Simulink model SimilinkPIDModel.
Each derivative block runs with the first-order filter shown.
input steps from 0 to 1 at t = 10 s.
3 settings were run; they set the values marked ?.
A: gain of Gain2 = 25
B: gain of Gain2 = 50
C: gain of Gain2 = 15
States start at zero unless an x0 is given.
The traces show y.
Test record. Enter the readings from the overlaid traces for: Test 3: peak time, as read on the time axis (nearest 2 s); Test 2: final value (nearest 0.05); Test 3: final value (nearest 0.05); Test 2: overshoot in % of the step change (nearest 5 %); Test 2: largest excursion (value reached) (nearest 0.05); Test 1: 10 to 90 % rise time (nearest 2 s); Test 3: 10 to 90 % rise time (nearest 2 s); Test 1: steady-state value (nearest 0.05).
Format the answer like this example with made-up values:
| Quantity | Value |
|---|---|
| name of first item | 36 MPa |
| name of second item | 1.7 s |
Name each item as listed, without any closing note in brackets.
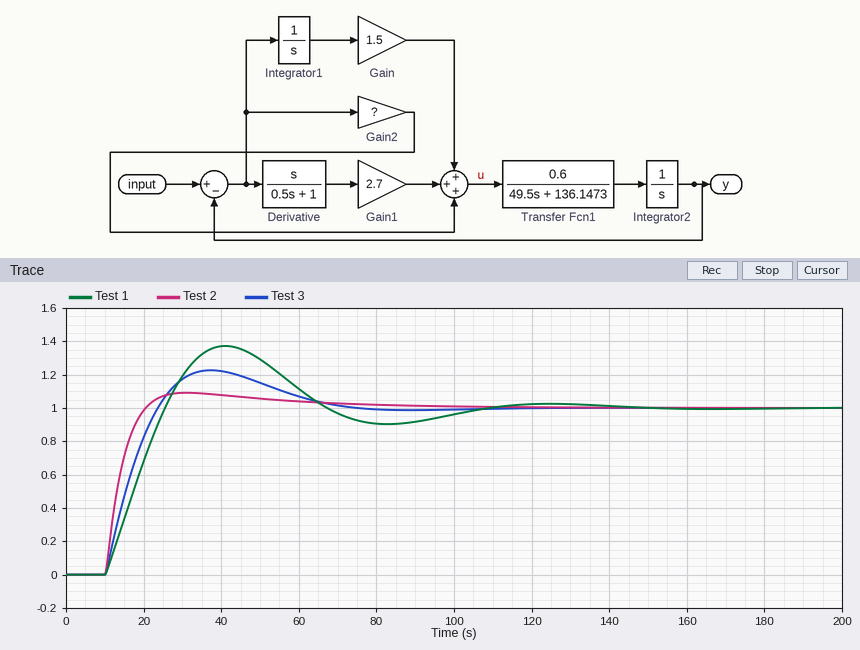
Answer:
| Quantity | Value |
|---|---|
| Test 3: peak time, as read on the time axis | 38 s |
| Test 2: final value | 1.00 |
| Test 3: final value | 1.00 |
| Test 2: overshoot in % of the step change | 10 % |
| Test 2: largest excursion (value reached) | 1.10 |
| Test 1: 10 to 90 % rise time | 12 s |
| Test 3: 10 to 90 % rise time | 10 s |
| Test 1: steady-state value | 1.00 |
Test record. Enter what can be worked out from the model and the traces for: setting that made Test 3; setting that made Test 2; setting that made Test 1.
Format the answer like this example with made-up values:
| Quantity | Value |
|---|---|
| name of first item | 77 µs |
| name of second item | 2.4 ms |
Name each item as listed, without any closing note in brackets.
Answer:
| Quantity | Value |
|---|---|
| setting that made Test 3 | A |
| setting that made Test 2 | B |
| setting that made Test 1 | C |
